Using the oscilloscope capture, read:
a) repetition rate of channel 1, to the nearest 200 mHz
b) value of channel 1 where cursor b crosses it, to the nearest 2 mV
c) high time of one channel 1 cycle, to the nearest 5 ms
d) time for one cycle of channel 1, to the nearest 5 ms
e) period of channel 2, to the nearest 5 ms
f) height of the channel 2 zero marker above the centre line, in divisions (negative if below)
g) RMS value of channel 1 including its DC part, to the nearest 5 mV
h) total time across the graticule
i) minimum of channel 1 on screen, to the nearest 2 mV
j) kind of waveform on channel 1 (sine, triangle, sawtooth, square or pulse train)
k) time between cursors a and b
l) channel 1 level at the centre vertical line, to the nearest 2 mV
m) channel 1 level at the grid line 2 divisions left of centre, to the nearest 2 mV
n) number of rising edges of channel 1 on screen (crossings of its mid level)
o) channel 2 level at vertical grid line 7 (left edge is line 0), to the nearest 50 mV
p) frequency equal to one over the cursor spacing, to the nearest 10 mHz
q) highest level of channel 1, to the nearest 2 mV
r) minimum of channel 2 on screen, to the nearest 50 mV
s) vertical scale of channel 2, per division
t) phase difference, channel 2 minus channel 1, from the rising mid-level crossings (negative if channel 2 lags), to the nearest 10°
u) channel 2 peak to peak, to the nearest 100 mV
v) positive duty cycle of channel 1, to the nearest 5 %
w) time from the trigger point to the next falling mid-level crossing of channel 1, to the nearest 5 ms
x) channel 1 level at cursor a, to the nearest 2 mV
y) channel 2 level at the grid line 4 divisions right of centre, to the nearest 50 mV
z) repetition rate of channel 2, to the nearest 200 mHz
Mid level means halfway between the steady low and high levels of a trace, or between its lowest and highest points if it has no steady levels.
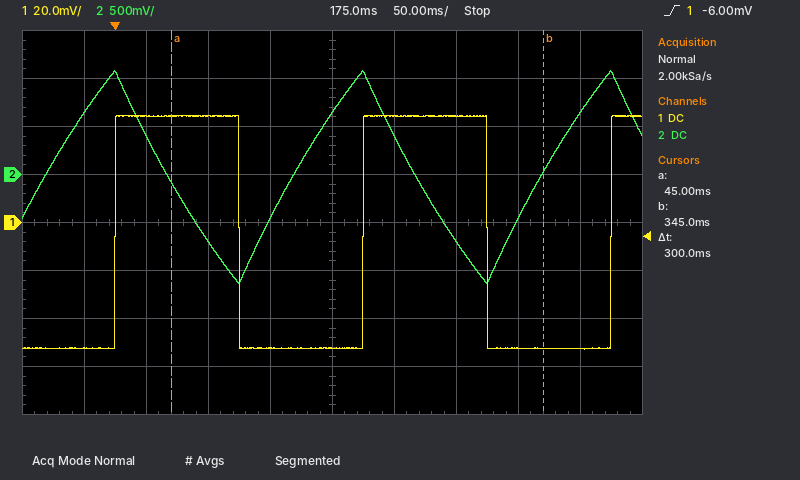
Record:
5.0 Hz
-52 mV
100 ms
200 ms
200 ms
+1.0 div
50 mV
500 ms
-52 mV
square
300 ms
-52 mV
44 mV
3
-700 mV
3.33 Hz
44 mV
-1.15 V
500 mV
+100°
2.20 V
50 %
100 ms
44 mV
650 mV
5.0 Hz
